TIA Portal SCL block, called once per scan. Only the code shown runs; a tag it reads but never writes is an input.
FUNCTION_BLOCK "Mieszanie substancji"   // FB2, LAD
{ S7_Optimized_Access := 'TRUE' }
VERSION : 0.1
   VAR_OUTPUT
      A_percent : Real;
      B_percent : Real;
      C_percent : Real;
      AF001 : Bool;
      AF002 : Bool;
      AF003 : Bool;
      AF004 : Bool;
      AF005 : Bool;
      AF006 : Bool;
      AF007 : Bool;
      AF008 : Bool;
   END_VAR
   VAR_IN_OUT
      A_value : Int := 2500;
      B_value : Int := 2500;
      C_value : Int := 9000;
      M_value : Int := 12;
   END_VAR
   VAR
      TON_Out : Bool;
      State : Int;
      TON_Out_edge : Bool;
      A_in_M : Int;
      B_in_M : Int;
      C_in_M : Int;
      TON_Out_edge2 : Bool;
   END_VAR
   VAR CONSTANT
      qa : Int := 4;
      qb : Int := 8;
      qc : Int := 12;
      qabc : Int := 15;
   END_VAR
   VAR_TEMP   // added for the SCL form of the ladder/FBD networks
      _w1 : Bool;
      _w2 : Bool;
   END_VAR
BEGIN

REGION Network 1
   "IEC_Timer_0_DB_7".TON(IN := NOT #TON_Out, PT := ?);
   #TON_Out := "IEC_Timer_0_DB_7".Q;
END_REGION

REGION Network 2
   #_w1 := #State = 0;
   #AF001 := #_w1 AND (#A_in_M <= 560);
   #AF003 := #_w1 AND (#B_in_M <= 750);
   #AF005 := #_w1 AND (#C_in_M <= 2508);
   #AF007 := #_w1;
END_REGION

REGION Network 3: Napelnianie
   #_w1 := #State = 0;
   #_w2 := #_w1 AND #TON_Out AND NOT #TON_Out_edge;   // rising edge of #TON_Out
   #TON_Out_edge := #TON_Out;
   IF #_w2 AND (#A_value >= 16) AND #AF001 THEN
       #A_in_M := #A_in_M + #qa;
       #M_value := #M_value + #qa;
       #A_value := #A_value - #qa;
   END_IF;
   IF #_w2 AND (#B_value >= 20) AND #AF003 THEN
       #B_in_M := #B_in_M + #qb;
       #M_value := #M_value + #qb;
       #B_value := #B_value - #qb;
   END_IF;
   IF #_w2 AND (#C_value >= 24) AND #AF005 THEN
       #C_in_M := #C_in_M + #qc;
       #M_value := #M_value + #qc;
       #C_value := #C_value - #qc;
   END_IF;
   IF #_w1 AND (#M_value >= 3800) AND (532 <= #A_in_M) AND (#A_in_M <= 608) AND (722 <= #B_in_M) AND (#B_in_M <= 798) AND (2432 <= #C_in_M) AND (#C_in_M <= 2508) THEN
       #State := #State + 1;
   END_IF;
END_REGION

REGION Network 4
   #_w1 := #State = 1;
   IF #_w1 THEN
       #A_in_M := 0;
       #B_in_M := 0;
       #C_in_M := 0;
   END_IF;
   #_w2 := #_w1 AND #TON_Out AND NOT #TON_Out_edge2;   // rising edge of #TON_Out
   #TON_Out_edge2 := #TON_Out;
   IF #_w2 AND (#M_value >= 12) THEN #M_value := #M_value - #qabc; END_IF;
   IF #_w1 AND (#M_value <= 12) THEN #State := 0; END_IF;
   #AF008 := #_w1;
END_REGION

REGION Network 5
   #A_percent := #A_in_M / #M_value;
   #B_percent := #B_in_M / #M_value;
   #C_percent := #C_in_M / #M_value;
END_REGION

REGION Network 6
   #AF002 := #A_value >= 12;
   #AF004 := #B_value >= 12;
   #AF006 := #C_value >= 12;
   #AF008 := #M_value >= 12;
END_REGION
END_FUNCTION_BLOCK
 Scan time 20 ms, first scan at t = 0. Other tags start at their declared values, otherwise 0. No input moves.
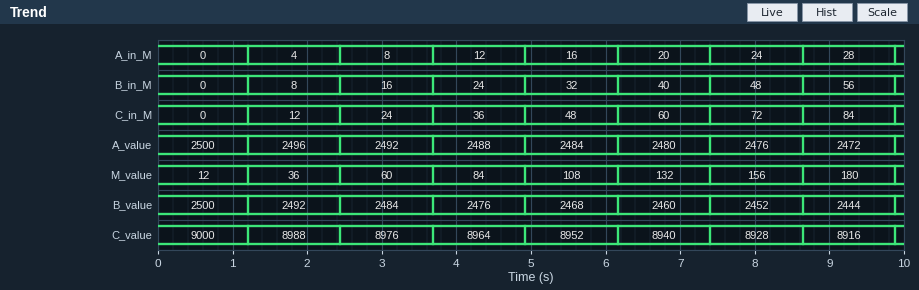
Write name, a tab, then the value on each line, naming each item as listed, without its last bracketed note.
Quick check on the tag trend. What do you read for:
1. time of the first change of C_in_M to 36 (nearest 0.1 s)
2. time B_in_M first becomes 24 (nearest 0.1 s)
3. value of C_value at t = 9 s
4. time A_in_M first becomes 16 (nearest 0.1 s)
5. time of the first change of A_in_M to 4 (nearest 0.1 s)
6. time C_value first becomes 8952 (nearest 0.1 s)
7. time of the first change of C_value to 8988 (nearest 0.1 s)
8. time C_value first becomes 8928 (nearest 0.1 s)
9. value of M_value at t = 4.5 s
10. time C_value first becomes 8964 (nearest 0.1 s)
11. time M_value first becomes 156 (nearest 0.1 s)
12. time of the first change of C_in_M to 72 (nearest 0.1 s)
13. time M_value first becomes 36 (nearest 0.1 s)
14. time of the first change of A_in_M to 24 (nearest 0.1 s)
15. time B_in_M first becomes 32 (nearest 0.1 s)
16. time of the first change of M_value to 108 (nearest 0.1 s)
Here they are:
time of the first change of C_in_M to 36	3.7 s
time B_in_M first becomes 24	3.7 s
value of C_value at t = 9 s	8916
time A_in_M first becomes 16	4.9 s
time of the first change of A_in_M to 4	1.2 s
time C_value first becomes 8952	4.9 s
time of the first change of C_value to 8988	1.2 s
time C_value first becomes 8928	7.4 s
value of M_value at t = 4.5 s	84
time C_value first becomes 8964	3.7 s
time M_value first becomes 156	7.4 s
time of the first change of C_in_M to 72	7.4 s
time M_value first becomes 36	1.2 s
time of the first change of A_in_M to 24	7.4 s
time B_in_M first becomes 32	4.9 s
time of the first change of M_value to 108	4.9 s
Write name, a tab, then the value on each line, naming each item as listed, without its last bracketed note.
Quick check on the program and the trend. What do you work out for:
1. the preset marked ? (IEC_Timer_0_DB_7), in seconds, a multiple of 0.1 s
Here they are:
the preset marked ? (IEC_Timer_0_DB_7), in seconds, a multiple of 0.1 s	1.2 s
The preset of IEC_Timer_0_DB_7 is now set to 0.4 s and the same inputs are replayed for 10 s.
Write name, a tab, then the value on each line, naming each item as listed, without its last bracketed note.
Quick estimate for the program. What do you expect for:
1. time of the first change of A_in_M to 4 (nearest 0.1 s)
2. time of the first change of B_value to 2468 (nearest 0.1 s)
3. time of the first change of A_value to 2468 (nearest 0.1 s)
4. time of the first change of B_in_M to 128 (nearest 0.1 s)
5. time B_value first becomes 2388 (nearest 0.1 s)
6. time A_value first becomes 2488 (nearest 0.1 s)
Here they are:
time of the first change of A_in_M to 4	0.4 s
time of the first change of B_value to 2468	1.7 s
time of the first change of A_value to 2468	3.5 s
time of the first change of B_in_M to 128	7.0 s
time B_value first becomes 2388	6.1 s
time A_value first becomes 2488	1.3 s
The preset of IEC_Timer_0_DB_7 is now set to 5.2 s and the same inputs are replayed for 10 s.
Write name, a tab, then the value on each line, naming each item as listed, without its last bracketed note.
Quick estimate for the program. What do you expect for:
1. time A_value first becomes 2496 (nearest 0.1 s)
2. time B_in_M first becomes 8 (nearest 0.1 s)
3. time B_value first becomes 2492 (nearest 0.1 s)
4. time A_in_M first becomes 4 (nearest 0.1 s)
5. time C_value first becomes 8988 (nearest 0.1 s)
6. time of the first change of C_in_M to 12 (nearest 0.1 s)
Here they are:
time A_value first becomes 2496	5.2 s
time B_in_M first becomes 8	5.2 s
time B_value first becomes 2492	5.2 s
time A_in_M first becomes 4	5.2 s
time C_value first becomes 8988	5.2 s
time of the first change of C_in_M to 12	5.2 s
